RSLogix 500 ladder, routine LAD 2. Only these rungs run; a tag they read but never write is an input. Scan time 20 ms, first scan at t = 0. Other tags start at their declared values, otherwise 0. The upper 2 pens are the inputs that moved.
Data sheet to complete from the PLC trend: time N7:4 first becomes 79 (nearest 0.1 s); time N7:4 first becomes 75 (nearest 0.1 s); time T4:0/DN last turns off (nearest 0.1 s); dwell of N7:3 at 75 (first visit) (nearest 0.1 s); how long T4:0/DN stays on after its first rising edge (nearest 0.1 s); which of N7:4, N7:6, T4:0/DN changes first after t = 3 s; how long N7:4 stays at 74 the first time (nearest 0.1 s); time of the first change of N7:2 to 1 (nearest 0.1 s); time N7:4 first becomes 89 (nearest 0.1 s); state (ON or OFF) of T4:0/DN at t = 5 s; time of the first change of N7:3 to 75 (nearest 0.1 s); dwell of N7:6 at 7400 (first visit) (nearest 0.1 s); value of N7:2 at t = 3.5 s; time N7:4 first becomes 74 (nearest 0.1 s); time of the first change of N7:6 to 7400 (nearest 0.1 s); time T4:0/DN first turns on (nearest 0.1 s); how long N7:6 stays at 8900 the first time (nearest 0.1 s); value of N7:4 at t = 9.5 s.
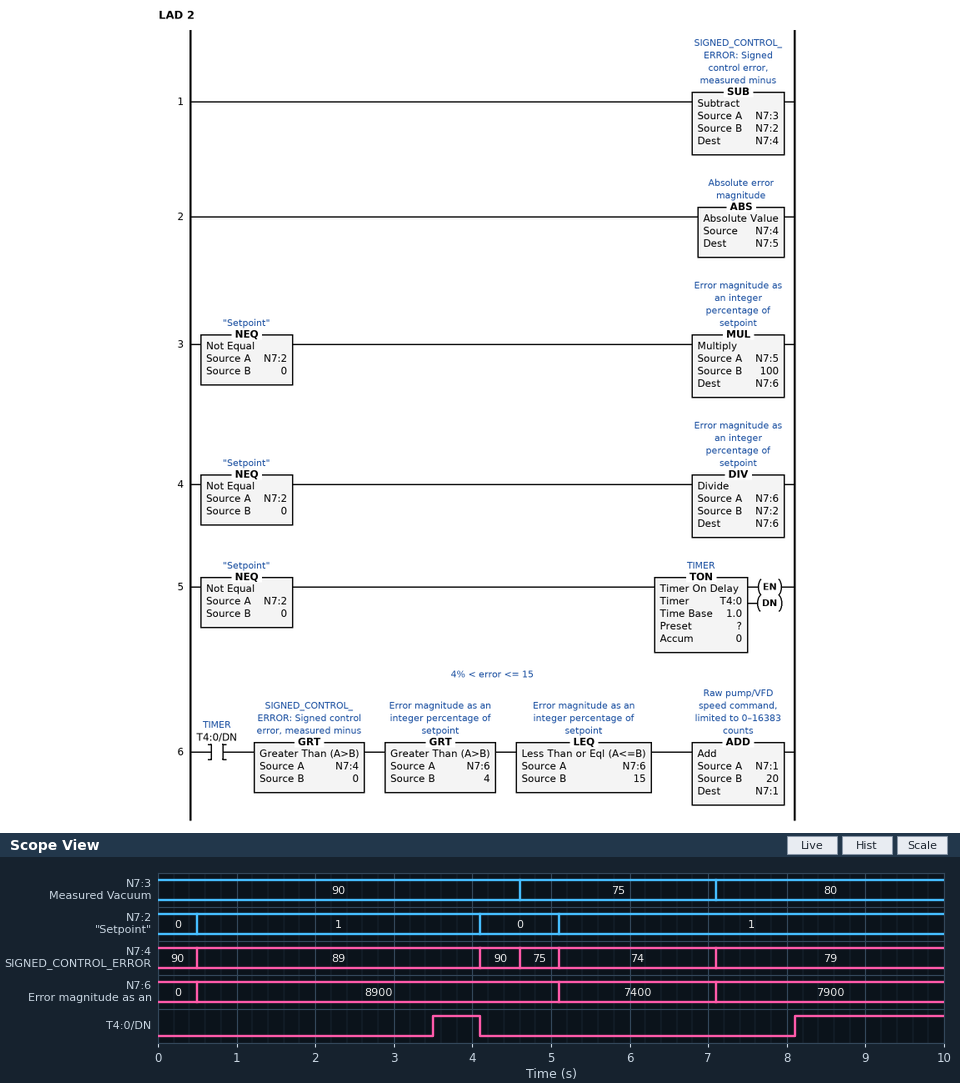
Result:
7.1 s
4.6 s
4.1 s
2.5 s
0.6 s
T4:0/DN
2.0 s
0.5 s
0.5 s
OFF
4.6 s
2.0 s
1
5.1 s
5.1 s
3.5 s
4.6 s
79
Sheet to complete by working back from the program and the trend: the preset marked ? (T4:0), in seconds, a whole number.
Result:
3 s
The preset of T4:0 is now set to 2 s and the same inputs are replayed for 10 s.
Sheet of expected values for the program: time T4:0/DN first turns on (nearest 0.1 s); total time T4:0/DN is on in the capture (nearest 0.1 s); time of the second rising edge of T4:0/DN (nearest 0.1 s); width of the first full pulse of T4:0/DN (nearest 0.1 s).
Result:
2.5 s
4.5 s
7.1 s
1.6 s
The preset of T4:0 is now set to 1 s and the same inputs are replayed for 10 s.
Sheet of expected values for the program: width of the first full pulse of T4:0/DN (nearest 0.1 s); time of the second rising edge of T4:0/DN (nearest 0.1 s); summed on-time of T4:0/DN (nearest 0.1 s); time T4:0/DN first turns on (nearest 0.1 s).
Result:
2.6 s
6.1 s
6.5 s
1.5 s
